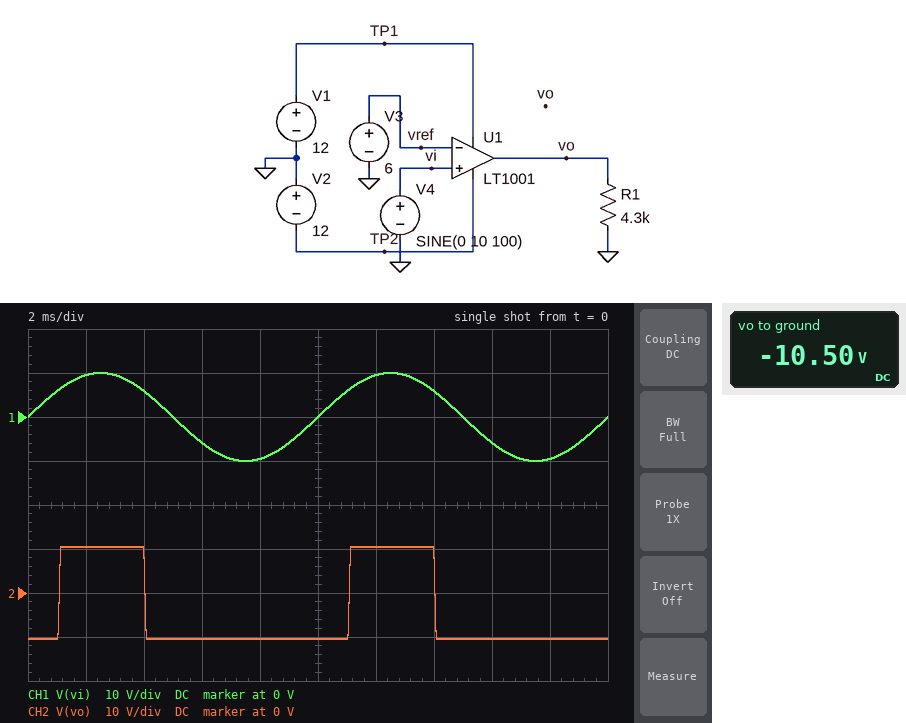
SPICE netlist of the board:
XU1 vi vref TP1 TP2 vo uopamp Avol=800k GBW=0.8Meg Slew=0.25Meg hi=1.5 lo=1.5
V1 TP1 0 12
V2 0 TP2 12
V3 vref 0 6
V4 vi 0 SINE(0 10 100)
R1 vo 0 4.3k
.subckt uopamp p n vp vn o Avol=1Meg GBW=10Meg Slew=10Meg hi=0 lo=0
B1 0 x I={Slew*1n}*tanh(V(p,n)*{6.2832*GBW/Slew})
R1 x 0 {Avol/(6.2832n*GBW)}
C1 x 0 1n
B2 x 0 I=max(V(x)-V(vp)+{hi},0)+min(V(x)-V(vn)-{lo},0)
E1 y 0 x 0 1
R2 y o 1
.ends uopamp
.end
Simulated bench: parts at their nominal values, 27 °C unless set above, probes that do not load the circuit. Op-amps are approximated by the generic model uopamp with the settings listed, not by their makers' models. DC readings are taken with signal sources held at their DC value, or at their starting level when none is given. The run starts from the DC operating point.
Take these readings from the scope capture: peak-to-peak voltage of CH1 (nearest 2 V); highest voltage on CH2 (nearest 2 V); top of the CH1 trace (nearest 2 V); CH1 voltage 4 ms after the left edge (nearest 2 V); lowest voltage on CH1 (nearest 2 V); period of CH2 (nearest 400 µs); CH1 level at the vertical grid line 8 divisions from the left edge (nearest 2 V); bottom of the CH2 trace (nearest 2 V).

20 V
10 V
10 V
6 V
-10 V
10.0 ms
-6 V
-10 V
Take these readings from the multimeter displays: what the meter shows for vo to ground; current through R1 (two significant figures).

-10.50 V
2.4 mA
